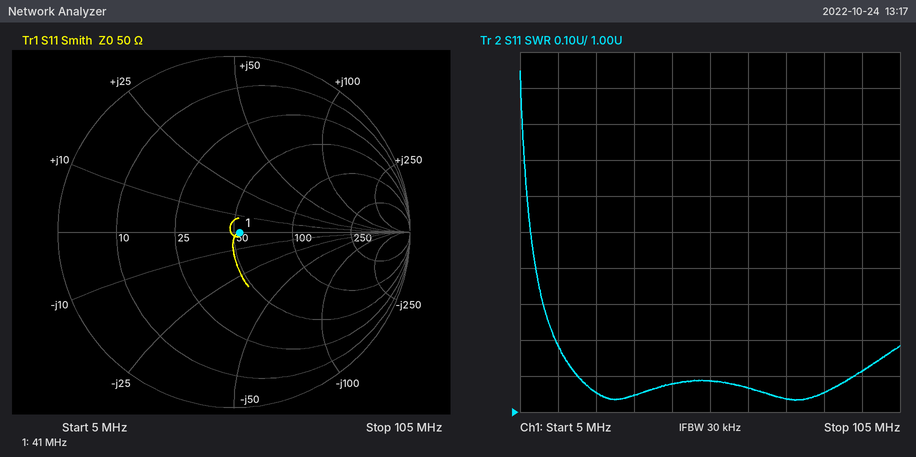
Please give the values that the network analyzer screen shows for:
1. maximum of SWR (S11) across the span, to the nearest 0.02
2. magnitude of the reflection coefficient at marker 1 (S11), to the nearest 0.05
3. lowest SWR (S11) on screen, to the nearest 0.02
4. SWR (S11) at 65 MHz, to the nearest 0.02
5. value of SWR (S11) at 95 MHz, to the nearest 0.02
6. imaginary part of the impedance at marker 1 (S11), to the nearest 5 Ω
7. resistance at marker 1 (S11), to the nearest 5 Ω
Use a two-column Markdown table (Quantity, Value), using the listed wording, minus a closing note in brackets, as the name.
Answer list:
| Quantity | Value |
|---|---|
| maximum of SWR (S11) across the span, to the nearest 0.02 | 1.94 |
| magnitude of the reflection coefficient at marker 1 (S11), to the nearest 0.05 | 0.05 |
| lowest SWR (S11) on screen, to the nearest 0.02 | 1.04 |
| SWR (S11) at 65 MHz, to the nearest 0.02 | 1.06 |
| value of SWR (S11) at 95 MHz, to the nearest 0.02 | 1.12 |
| imaginary part of the impedance at marker 1 (S11), to the nearest 5 Ω | 0 Ω |
| resistance at marker 1 (S11), to the nearest 5 Ω | 55 Ω |
